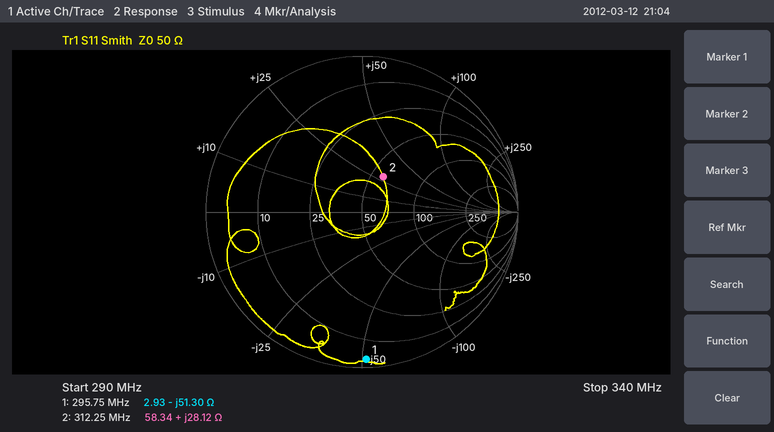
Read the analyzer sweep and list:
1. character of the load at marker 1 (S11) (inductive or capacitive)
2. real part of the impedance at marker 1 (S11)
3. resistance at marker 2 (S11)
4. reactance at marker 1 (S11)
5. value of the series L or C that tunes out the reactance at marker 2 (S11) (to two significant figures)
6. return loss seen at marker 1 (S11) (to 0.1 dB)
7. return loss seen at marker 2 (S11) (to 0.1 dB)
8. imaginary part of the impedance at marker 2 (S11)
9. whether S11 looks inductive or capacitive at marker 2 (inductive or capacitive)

capacitive
2.93 Ω
58.34 Ω
-51.30 Ω
18 pF
0.5 dB
11.6 dB
+28.12 Ω
inductive
